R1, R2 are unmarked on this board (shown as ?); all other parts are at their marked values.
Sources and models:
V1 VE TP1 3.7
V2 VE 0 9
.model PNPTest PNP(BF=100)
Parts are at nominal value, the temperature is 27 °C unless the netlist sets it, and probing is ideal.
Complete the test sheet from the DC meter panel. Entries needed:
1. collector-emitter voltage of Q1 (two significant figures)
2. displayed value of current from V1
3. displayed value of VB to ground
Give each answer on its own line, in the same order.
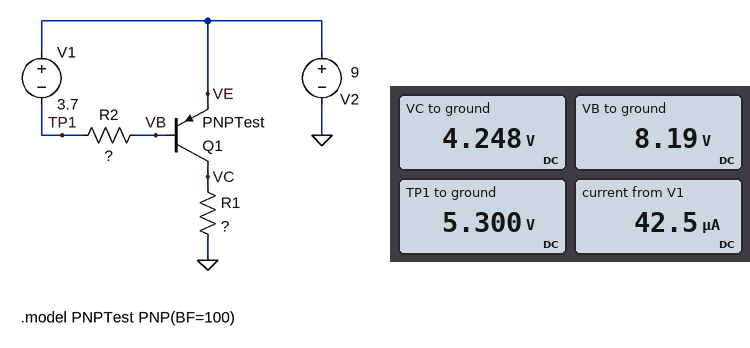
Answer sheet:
-4.8 V
42.5 µA
8.19 V
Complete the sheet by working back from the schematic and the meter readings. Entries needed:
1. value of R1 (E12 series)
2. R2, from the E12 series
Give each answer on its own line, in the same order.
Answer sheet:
1 kΩ
68 kΩ
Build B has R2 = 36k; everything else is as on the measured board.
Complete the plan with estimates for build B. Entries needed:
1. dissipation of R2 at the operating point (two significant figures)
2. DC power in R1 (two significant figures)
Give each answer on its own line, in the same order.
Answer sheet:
230 µW
64 mW
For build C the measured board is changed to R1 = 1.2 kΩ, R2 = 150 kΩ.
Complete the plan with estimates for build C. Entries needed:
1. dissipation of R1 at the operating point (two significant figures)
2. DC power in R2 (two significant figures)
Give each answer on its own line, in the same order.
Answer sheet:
4.5 mW
56 µW
